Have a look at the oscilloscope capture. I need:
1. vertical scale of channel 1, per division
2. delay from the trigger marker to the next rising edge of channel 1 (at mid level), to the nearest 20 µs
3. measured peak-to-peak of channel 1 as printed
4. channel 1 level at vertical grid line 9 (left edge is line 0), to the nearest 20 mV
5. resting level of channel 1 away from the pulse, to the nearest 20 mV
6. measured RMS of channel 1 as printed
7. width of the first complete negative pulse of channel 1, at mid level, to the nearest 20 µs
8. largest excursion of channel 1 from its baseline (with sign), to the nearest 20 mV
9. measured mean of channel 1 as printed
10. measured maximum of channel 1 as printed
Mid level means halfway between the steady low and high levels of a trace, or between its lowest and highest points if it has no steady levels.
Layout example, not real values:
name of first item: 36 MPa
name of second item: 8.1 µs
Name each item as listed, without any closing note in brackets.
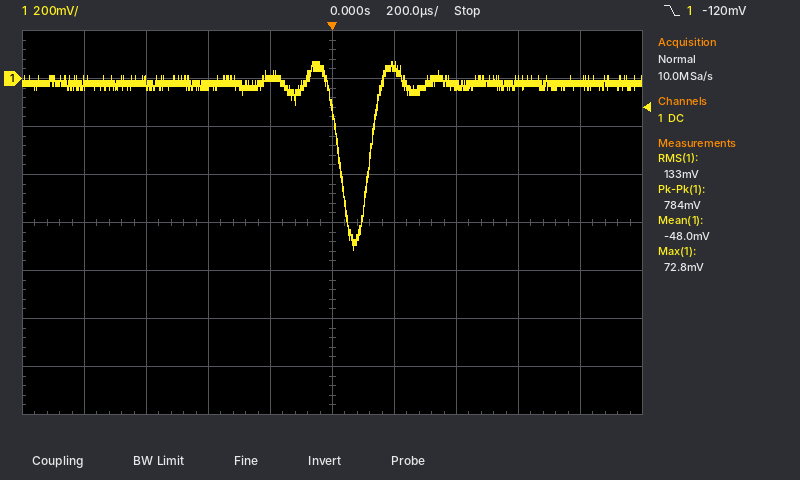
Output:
vertical scale of channel 1, per division: 200 mV
delay from the trigger marker to the next rising edge of channel 1 (at mid level), to the nearest 20 µs: 120 µs
measured peak-to-peak of channel 1 as printed: 784 mV
channel 1 level at vertical grid line 9 (left edge is line 0), to the nearest 20 mV: -20 mV
resting level of channel 1 away from the pulse, to the nearest 20 mV: -20 mV
measured RMS of channel 1 as printed: 133 mV
width of the first complete negative pulse of channel 1, at mid level, to the nearest 20 µs: 100 µs
largest excursion of channel 1 from its baseline (with sign), to the nearest 20 mV: -700 mV
measured mean of channel 1 as printed: -48.0 mV
measured maximum of channel 1 as printed: 72.8 mV
